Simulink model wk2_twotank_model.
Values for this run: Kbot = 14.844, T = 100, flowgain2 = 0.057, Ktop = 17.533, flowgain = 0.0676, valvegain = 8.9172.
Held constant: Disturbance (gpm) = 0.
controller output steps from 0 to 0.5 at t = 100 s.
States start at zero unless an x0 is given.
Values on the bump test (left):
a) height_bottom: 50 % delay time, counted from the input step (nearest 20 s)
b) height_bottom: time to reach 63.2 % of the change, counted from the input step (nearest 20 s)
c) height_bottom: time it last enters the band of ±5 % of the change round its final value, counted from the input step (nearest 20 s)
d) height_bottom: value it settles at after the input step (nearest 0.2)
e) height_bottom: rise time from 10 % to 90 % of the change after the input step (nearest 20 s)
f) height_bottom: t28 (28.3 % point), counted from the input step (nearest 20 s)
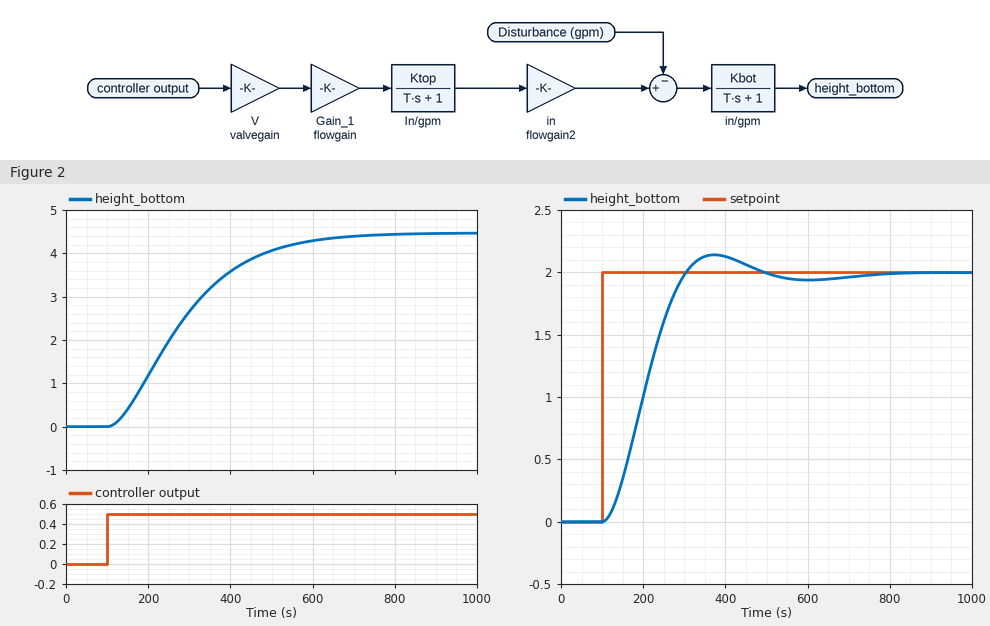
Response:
160 s
220 s
480 s
4.4
340 s
100 s
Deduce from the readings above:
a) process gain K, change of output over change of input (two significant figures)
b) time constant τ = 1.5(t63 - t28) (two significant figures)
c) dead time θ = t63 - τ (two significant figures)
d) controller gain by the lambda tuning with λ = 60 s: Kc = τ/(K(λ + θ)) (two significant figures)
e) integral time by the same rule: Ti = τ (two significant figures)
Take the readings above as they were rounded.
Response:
8.8
180 s
40 s
0.20
180 s
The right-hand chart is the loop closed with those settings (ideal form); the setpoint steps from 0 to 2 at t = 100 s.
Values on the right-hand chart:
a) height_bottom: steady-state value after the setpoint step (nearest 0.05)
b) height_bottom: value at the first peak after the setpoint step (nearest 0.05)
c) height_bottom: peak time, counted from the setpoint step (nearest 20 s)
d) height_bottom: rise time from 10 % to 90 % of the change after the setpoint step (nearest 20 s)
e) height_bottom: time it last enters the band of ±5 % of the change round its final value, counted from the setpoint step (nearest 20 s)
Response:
2.00
2.15
280 s
140 s
320 s
